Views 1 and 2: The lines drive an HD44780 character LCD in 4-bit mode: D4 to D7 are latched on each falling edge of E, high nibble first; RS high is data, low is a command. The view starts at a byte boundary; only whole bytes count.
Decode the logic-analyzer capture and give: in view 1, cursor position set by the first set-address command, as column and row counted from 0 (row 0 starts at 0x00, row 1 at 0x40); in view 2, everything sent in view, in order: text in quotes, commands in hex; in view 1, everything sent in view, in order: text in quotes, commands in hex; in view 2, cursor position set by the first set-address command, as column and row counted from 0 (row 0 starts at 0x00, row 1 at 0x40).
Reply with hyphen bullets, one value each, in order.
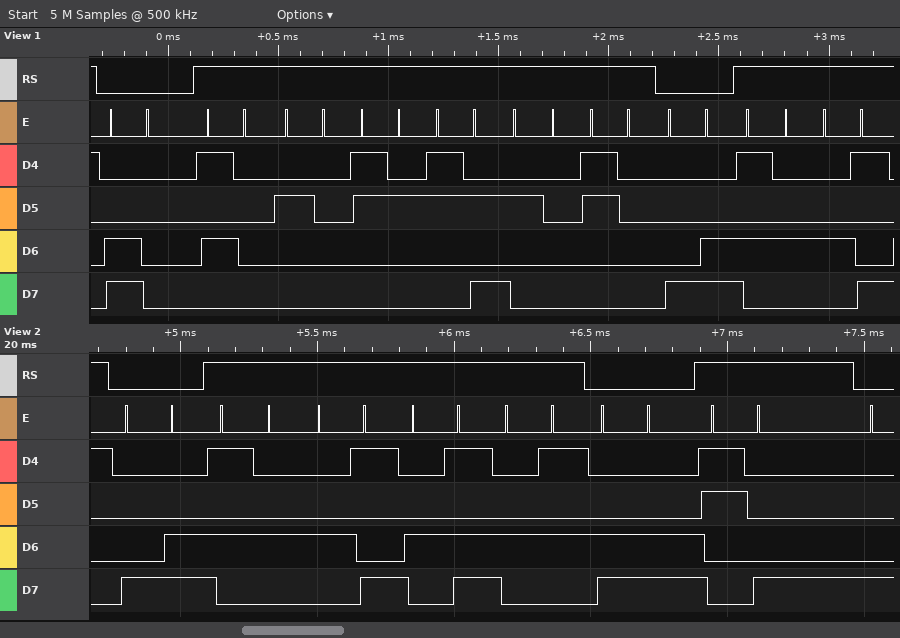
- column 0, row 1
- 0x8C "TIME" 0xCC "8"
- 0xC0 "P 2: 0" 0x8C "TI"
- column 12, row 0
